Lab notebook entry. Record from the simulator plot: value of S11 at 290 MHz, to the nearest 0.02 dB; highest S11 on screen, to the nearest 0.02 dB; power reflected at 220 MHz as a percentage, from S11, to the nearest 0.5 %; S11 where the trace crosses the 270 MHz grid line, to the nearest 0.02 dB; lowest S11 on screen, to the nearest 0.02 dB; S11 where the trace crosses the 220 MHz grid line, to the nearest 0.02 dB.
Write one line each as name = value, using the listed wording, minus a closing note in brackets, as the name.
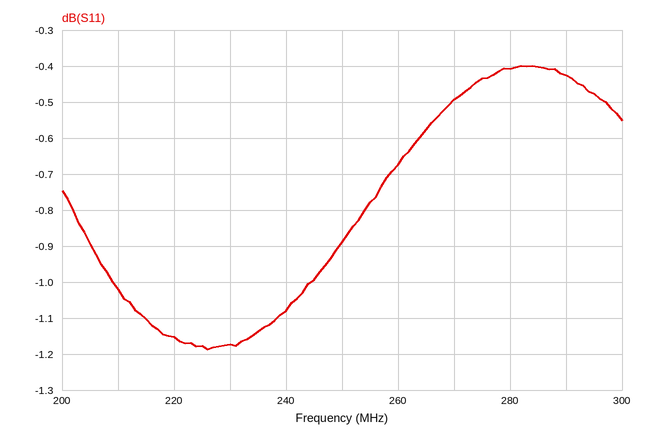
value of S11 at 290 MHz, to the nearest 0.02 dB = -0.42 dB
highest S11 on screen, to the nearest 0.02 dB = -0.40 dB
power reflected at 220 MHz as a percentage, from S11, to the nearest 0.5 % = 76.5 %
S11 where the trace crosses the 270 MHz grid line, to the nearest 0.02 dB = -0.50 dB
lowest S11 on screen, to the nearest 0.02 dB = -1.18 dB
S11 where the trace crosses the 220 MHz grid line, to the nearest 0.02 dB = -1.16 dB
